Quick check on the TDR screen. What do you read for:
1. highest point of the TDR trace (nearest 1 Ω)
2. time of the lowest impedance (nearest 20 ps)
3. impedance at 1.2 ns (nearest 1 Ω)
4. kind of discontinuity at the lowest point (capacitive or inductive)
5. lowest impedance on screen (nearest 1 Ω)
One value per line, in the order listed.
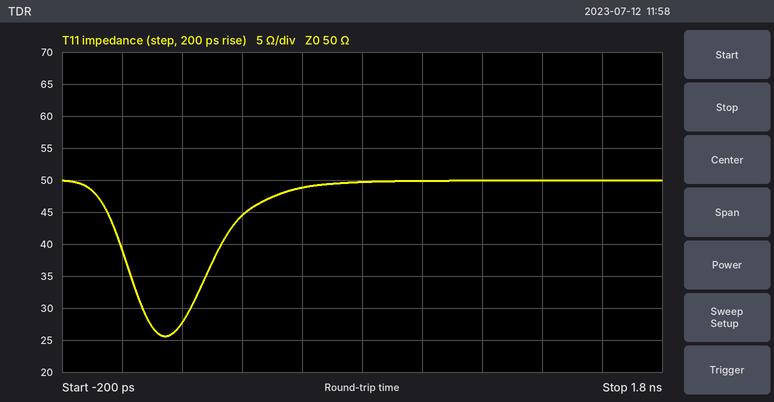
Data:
50 Ω
140 ps
50 Ω
capacitive
26 Ω
